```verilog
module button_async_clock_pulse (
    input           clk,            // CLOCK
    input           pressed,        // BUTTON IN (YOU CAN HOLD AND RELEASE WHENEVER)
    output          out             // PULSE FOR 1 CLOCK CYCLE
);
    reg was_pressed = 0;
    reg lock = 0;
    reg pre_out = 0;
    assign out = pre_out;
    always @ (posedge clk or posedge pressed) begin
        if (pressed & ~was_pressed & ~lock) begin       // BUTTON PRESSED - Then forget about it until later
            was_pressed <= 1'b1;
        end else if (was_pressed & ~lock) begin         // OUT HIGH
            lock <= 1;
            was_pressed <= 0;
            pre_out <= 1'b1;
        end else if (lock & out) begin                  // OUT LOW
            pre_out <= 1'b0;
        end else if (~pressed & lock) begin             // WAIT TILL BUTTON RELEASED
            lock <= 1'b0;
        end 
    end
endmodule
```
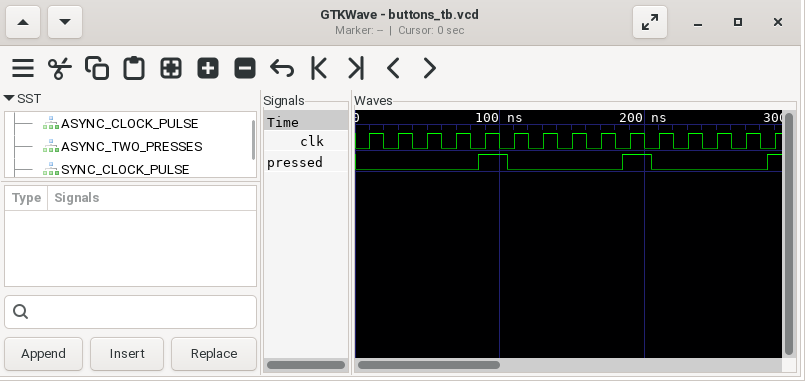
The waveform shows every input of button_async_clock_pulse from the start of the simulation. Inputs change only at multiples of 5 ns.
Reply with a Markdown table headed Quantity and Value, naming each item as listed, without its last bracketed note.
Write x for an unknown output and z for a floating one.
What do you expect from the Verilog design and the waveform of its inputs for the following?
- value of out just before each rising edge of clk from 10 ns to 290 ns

| Quantity | Value |
|---|---|
| value of out just before each rising edge of clk from 10 ns to 290 ns | 0 0 0 0 0 1 0 0 0 0 1 0 0 0 0 |
